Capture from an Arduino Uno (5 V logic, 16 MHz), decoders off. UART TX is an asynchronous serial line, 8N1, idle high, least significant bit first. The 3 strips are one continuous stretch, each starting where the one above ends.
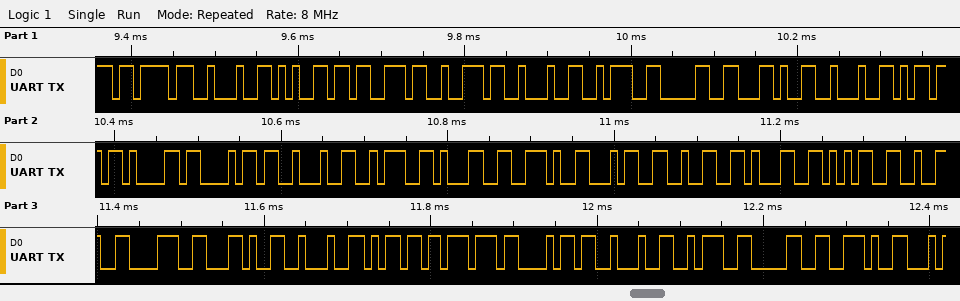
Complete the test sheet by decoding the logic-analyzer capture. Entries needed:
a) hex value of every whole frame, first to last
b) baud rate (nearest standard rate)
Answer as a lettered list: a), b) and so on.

a) 0x7B 0x22 0x65 0x73 0x72 0x22 0x3A 0x30 0x2C 0x22 0x6D 0x61 0x68 0x22 0x3A 0x31 0x2E 0x34 0x32 0x31 0x35 0x32 0x38 0x2C 0x22 0x6D 0x77 0x68 0x22 0x3A 0x30 0x2E
b) 115200 baud
